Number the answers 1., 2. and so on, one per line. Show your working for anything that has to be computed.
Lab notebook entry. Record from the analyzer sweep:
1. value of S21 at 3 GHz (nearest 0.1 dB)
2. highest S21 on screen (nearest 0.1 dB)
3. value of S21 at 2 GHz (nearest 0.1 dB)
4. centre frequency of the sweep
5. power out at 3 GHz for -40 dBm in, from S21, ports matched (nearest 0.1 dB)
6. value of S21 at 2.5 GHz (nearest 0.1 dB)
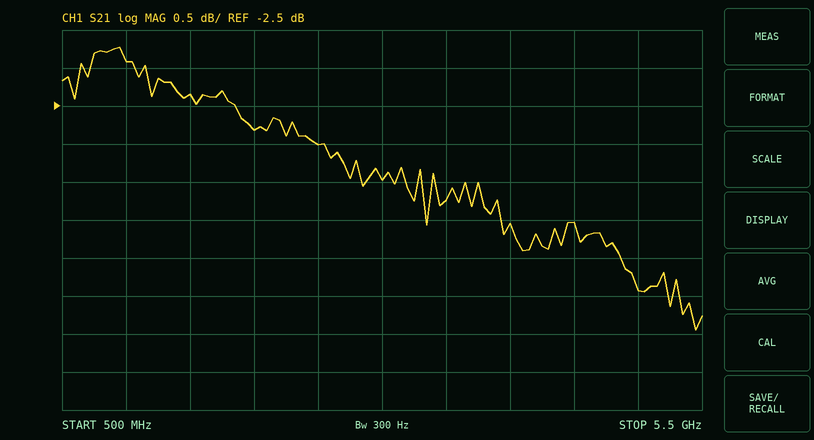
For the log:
1. -3.5 dB
2. -1.7 dB
3. -2.8 dB
4. 3 GHz
5. -40 dBm + (-3.5 dB) = -43.5 dBm
6. -3.0 dB
